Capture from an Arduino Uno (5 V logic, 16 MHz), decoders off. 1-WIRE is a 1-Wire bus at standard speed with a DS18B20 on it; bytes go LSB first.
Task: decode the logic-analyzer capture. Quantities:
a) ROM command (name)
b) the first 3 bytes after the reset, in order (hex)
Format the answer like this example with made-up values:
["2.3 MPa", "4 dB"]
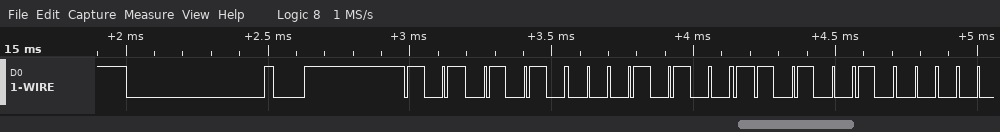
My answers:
["Match ROM", "55 28 4B"]
